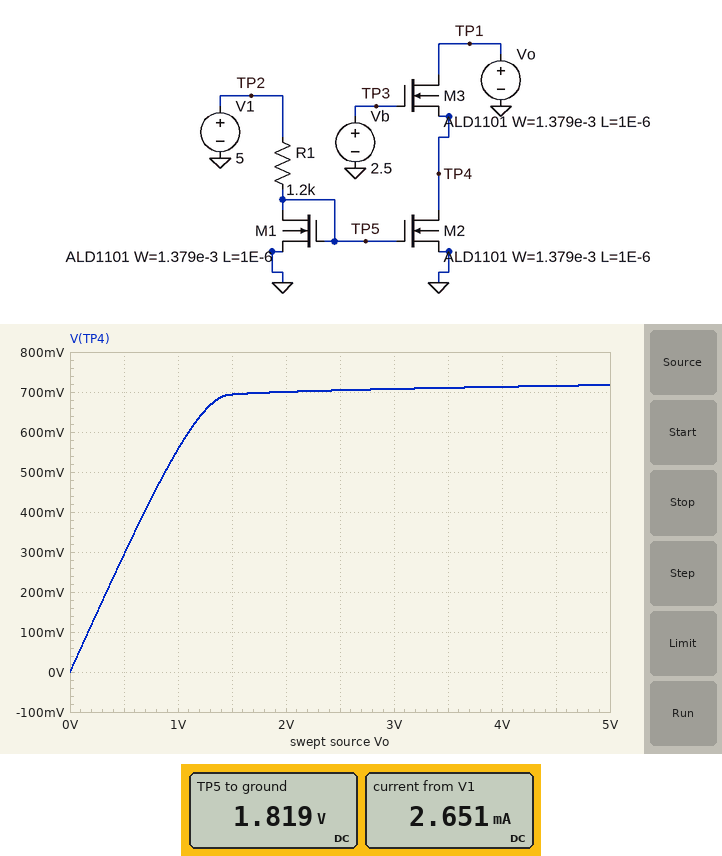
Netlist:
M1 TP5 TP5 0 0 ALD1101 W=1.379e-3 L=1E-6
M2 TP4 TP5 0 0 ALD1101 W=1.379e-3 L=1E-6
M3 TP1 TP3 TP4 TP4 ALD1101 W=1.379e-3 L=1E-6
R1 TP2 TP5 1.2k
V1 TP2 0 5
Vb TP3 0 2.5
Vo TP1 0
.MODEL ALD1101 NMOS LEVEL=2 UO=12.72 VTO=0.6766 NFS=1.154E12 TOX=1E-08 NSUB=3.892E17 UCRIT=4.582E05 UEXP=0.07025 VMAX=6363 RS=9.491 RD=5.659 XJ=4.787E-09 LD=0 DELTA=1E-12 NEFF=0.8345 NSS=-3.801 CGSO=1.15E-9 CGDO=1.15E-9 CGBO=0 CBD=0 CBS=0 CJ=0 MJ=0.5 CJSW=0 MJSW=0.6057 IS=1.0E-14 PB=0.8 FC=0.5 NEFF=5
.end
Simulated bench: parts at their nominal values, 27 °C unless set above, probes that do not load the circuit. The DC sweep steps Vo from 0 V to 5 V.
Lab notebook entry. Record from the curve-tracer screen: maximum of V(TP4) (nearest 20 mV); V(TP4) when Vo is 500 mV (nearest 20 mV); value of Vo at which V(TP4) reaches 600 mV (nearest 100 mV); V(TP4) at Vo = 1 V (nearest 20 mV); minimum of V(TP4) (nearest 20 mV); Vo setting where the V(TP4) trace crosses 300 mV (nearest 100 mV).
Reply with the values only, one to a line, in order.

720 mV
300 mV
1.1 V
560 mV
0 V
500 mV
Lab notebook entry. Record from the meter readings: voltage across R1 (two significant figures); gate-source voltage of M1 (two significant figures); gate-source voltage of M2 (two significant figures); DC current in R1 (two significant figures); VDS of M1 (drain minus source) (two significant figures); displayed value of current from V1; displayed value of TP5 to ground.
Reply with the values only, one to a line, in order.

3.2 V
1.8 V
1.8 V
2.7 mA
1.8 V
2.651 mA
1.819 V
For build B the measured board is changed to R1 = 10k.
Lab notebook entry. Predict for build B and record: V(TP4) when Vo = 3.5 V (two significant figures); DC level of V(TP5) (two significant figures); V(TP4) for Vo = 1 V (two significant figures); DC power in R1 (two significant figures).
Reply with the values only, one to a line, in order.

1.4 V
1.1 V
920 mV
1.5 mW
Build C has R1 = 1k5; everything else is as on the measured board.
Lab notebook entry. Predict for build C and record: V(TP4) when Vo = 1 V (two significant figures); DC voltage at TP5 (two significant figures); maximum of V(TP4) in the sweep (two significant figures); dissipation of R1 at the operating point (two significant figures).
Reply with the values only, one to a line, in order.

600 mV
1.7 V
810 mV
7.2 mW
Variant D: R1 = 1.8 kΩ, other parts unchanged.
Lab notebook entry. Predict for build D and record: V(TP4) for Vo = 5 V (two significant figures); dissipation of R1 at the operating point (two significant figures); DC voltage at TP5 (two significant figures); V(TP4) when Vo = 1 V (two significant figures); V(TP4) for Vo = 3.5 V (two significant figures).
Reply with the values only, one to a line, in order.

890 mV
6.3 mW
1.6 V
650 mV
880 mV
